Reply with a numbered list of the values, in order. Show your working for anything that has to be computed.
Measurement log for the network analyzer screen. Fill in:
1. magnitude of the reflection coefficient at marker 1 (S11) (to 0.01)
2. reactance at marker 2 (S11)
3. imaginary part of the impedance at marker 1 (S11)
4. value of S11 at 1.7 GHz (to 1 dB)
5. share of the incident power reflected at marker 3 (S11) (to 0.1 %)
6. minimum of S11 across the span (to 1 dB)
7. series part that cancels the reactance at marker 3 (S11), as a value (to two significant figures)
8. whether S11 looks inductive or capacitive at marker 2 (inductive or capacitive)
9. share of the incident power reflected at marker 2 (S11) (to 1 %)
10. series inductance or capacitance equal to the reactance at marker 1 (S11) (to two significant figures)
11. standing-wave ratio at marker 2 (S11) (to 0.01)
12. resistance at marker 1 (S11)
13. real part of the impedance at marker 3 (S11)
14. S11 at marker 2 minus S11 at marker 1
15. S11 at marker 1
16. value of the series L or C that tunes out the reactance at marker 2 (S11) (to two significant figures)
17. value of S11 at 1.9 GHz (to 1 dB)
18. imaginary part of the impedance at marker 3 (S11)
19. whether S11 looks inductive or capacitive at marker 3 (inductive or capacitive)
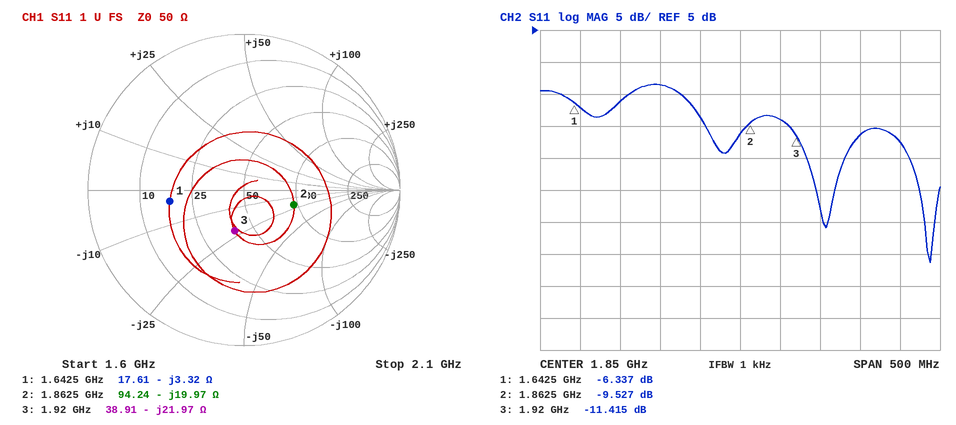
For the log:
1. 10^(-6.337/20) ≈ 0.48
2. -19.97 Ω
3. -3.32 Ω
4. -6 dB
5. 10^(-11.415/10) ≈ 7.2 %
6. -31 dB
7. L = 21.97 Ω/(2π × 1.92 GHz) ≈ 1.8 nH
8. capacitive
9. 10^(-9.527/10) ≈ 11 %
10. C = 1/(2π × 1.6425 GHz × 3.32 Ω) ≈ 29 pF
11. 2.00
12. 17.61 Ω
13. 38.91 Ω
14. -9.527 − (-6.337) = -3.190 dB
15. -6.337 dB
16. L = 19.97 Ω/(2π × 1.8625 GHz) ≈ 1.7 nH
17. -9 dB
18. -21.97 Ω
19. capacitive
